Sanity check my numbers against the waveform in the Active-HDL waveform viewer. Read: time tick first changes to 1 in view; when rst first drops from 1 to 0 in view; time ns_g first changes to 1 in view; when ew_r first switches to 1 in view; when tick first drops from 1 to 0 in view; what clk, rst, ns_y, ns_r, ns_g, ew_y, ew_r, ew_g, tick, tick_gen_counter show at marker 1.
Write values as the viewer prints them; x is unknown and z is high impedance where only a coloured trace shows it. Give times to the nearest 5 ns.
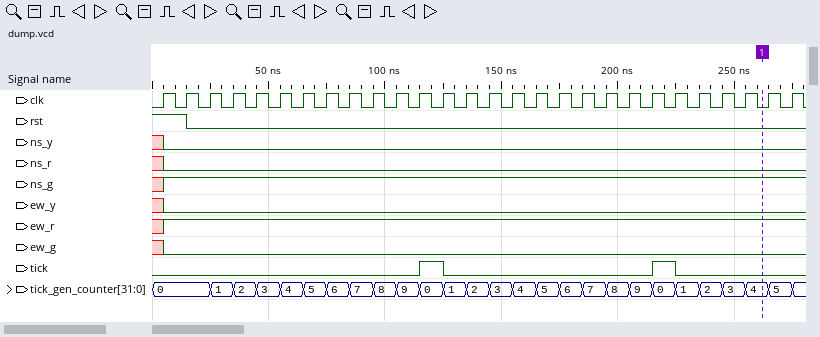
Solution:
115 ns
15 ns
5 ns
5 ns
125 ns
clk=0, rst=0, ns_y=0, ns_r=0, ns_g=1, ew_y=0, ew_r=1, ew_g=0, tick=0, tick_gen_counter=4
